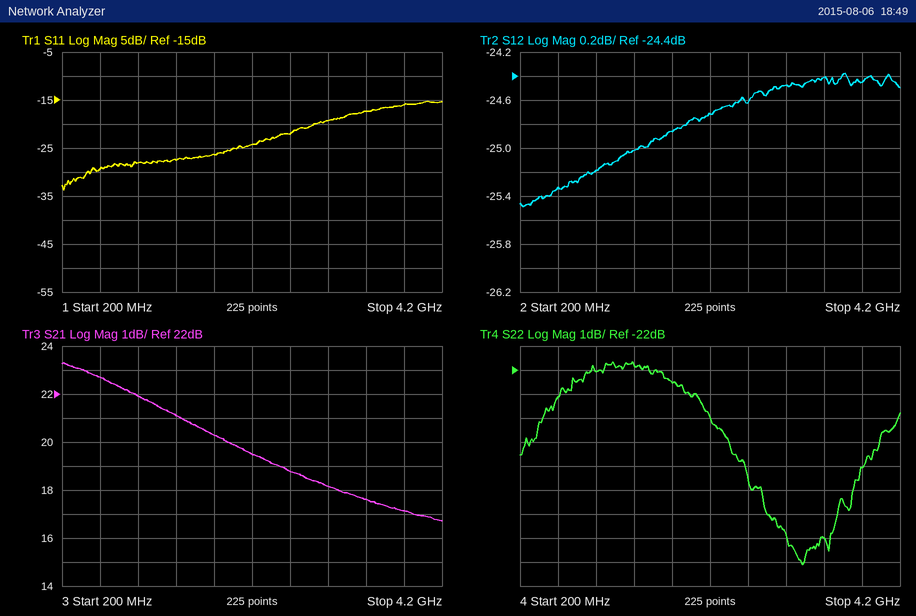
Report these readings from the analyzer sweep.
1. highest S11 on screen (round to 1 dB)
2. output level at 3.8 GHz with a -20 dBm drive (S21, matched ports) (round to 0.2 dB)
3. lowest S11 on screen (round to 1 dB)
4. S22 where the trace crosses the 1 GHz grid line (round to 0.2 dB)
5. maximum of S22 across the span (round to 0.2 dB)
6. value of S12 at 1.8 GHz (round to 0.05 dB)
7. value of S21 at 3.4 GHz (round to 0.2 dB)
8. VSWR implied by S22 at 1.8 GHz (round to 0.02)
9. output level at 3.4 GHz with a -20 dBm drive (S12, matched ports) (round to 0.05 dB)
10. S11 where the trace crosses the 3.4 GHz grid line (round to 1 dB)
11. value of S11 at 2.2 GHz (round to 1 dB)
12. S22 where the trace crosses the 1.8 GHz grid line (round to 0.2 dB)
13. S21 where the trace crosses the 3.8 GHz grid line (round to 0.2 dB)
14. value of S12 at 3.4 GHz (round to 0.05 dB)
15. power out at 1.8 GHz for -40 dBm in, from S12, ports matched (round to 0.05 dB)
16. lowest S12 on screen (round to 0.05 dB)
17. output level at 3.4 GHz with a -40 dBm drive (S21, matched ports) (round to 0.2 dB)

-15 dB
-2.8 dBm
-34 dB
-22.0 dB
-21.6 dB
-24.85 dB
17.6 dB
1.16
-44.40 dBm
-17 dB
-24 dB
-22.6 dB
17.2 dB
-24.40 dB
-64.85 dBm
-25.50 dB
-22.4 dBm
